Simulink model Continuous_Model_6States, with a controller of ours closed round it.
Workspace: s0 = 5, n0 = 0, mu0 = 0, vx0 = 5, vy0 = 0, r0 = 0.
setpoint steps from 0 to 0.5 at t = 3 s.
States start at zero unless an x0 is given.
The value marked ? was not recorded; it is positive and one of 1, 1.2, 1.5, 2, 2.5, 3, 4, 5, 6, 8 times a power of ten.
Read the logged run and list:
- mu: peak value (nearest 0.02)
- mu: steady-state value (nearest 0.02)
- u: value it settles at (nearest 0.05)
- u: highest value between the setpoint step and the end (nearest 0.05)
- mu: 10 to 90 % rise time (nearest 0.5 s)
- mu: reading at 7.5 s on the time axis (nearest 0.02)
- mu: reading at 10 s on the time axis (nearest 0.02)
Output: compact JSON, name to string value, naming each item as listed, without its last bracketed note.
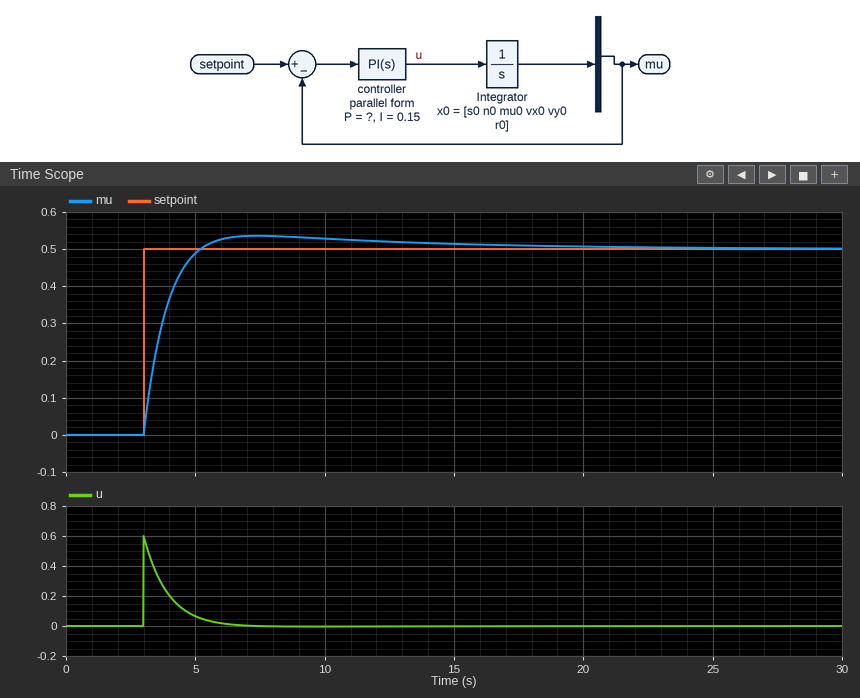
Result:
{"mu: peak value": "0.54", "mu: steady-state value": "0.50", "u: value it settles at": "0.00", "u: highest value between the setpoint step and the end": "0.60", "mu: 10 to 90 % rise time": "1.5 s", "mu: reading at 7.5 s on the time axis": "0.54", "mu: reading at 10 s on the time axis": "0.52"}
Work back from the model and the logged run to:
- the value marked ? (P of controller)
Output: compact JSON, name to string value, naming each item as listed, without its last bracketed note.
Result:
{"the value marked ?": "1.2"}
